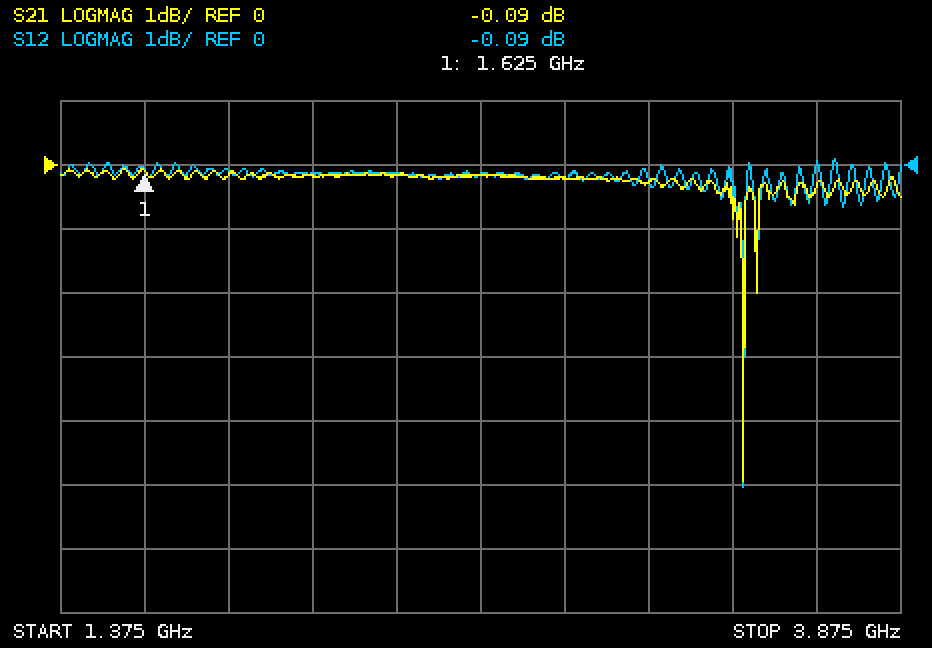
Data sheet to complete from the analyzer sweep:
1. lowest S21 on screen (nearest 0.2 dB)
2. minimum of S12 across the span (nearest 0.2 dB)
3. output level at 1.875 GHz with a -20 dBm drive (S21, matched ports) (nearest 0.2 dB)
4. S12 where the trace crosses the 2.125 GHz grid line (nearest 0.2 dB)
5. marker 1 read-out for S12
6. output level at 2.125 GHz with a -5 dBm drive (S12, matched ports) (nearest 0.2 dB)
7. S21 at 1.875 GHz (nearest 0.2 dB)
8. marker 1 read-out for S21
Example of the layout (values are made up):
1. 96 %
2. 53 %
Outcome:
1. -5.0 dB
2. -5.0 dB
3. -20.2 dBm
4. -0.2 dB
5. -0.09 dB
6. -5.2 dBm
7. -0.2 dB
8. -0.09 dB
